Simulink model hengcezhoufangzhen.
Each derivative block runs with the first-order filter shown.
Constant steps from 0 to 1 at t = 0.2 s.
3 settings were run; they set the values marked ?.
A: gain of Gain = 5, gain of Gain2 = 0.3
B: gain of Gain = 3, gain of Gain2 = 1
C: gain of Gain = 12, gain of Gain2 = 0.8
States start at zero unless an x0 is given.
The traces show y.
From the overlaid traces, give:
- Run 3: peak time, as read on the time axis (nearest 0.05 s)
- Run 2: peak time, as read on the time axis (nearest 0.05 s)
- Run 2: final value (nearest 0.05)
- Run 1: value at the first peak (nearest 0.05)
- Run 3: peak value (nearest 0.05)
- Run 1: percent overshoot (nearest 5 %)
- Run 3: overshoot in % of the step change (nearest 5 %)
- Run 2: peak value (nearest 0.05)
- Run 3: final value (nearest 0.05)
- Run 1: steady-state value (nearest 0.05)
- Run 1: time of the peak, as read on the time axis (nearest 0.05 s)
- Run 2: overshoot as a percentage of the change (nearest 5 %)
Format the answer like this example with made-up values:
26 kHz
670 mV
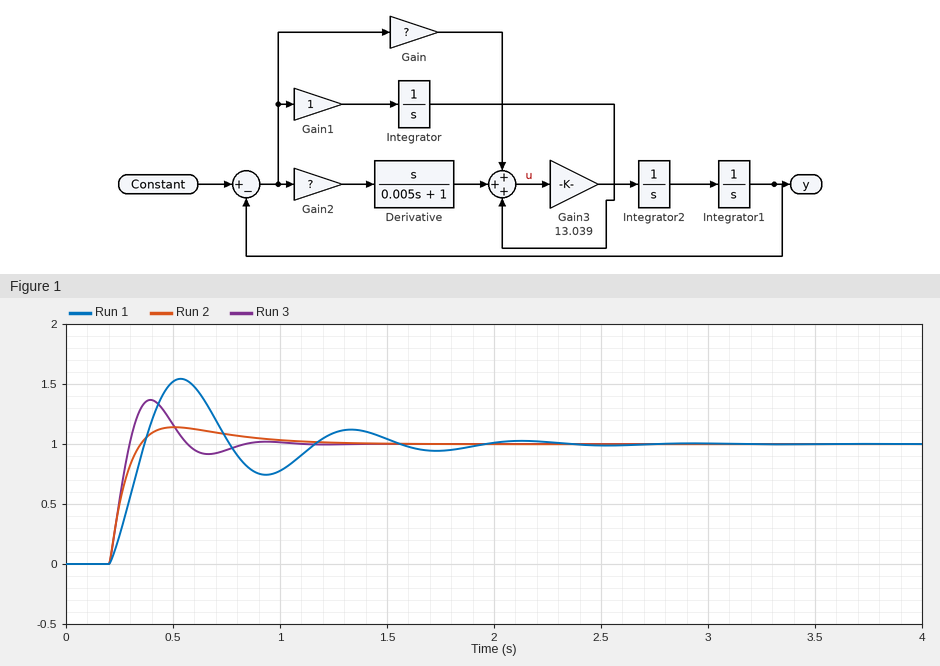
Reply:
0.40 s
0.50 s
1.00
1.55
1.35
55 %
35 %
1.15
1.00
1.00
0.55 s
15 %
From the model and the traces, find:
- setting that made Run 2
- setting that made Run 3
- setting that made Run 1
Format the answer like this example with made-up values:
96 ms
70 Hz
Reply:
B
C
A
